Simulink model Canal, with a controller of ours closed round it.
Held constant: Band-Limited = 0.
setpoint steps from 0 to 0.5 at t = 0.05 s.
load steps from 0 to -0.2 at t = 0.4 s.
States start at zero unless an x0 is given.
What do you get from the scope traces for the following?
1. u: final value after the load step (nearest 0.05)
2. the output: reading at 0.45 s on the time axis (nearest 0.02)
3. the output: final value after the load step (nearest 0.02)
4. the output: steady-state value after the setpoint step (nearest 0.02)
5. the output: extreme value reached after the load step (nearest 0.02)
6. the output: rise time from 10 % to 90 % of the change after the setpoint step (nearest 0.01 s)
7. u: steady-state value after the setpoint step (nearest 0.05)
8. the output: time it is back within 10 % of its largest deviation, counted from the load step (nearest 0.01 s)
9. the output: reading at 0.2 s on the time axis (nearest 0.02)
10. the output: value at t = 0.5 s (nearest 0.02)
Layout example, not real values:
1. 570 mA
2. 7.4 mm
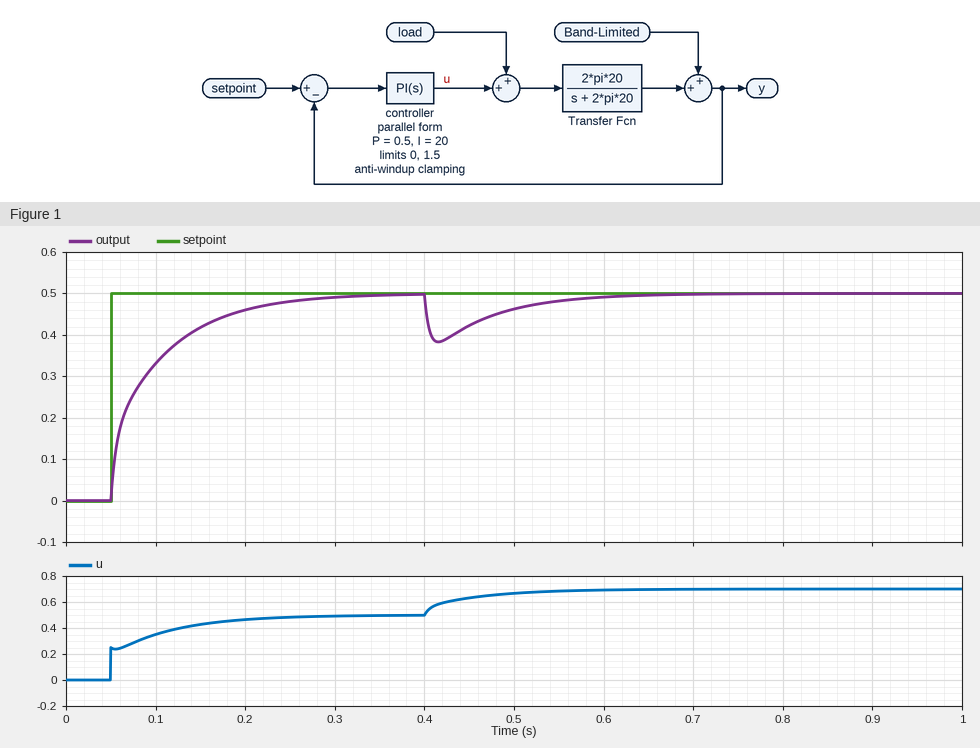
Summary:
1. 0.70
2. 0.42
3. 0.50
4. 0.50
5. 0.38
6. 0.13 s
7. 0.50
8. 0.18 s
9. 0.46
10. 0.46
